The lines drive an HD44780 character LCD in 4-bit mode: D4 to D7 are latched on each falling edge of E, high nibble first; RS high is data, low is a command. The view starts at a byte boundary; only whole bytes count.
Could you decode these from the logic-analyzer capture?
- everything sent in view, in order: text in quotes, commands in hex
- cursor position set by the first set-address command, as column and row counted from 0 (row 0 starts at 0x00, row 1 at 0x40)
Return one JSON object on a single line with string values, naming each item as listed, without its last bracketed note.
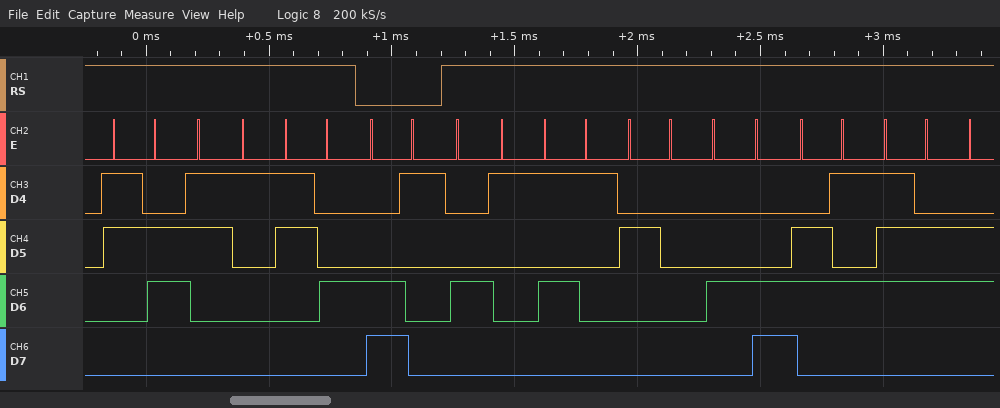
{"everything sent in view, in order: text in quotes, commands in hex": "\"614\" 0xC1 \"AQ Lev\"", "cursor position set by the first set-address command, as column and row counted from 0": "column 1, row 1"}
